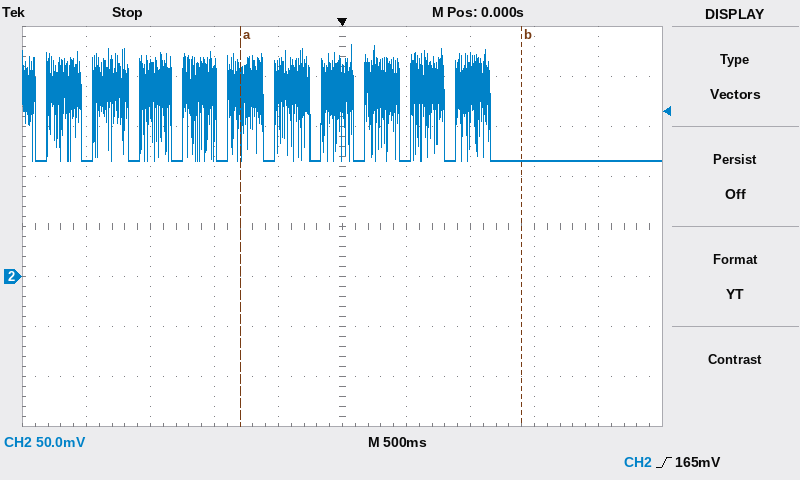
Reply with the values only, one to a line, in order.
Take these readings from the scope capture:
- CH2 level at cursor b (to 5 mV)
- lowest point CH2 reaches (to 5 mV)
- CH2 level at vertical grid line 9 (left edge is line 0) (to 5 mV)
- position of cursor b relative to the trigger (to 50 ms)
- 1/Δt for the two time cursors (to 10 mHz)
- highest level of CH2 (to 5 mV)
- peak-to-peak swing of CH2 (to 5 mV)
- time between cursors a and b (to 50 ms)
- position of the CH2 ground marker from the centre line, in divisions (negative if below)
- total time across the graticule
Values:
115 mV
115 mV
115 mV
+1.40 s
450 mHz
230 mV
115 mV
2.20 s
-1.0 div
5 s
